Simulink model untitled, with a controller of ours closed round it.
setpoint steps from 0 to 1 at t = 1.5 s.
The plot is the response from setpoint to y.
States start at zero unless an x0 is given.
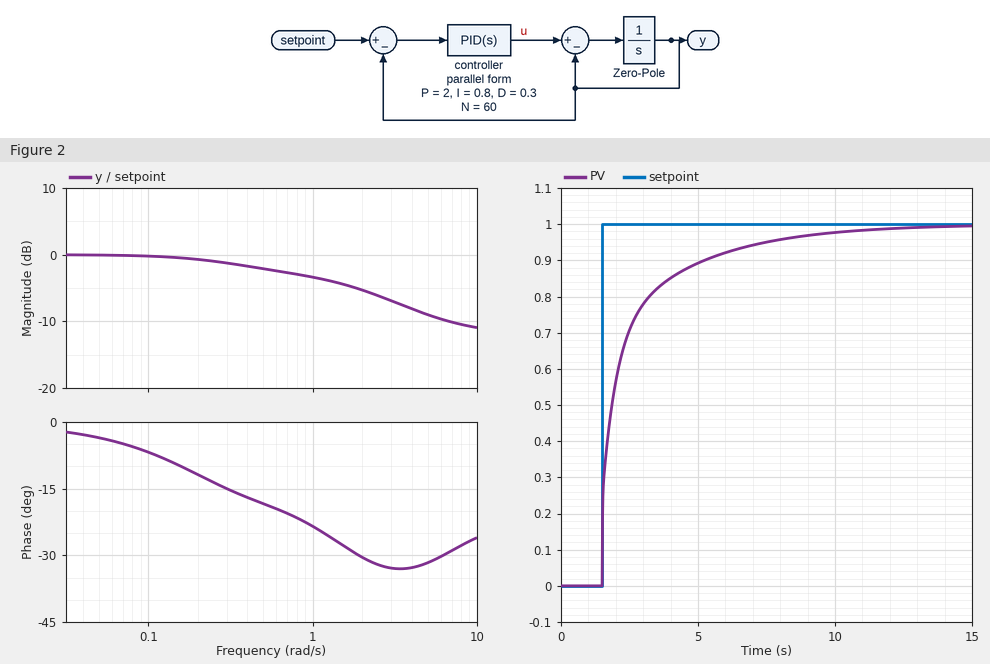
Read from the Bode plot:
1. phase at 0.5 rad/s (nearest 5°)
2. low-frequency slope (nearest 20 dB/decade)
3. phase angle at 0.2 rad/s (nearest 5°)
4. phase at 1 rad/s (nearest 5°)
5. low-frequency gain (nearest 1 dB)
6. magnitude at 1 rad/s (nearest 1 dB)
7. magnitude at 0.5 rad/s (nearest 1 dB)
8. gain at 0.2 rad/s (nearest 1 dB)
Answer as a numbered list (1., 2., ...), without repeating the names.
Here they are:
1. -20°
2. 0 dB/decade
3. -10°
4. -25°
5. 0 dB
6. -3 dB
7. -2 dB
8. -1 dB
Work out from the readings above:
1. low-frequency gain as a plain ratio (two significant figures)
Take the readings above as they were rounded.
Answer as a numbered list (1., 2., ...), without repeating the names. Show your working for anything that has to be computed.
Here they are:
1. 10^(0 / 20) = 1.0
